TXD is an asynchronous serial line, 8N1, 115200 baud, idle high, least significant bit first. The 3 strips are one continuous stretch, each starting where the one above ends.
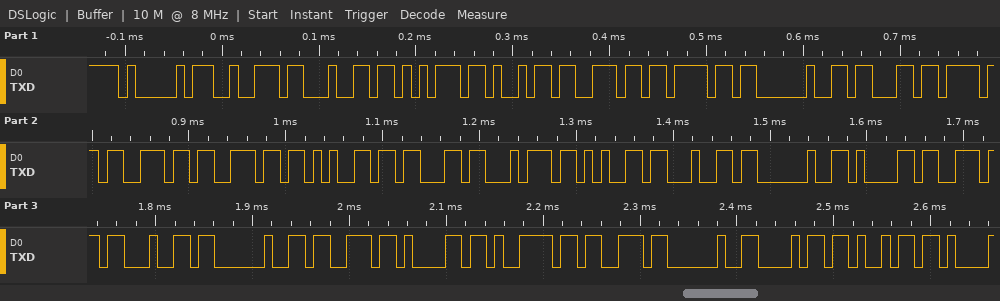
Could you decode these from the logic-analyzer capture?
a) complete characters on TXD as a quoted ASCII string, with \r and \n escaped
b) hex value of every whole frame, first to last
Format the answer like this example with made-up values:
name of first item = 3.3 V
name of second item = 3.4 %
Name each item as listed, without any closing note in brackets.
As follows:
complete characters on TXD as a quoted ASCII string, with \r and \n escaped = "Arduino connected and says hi"
hex value of every whole frame, first to last = 41 72 64 75 69 6E 6F 20 63 6F 6E 6E 65 63 74 65 64 20 61 6E 64 20 73 61 79 73 20 68 69
